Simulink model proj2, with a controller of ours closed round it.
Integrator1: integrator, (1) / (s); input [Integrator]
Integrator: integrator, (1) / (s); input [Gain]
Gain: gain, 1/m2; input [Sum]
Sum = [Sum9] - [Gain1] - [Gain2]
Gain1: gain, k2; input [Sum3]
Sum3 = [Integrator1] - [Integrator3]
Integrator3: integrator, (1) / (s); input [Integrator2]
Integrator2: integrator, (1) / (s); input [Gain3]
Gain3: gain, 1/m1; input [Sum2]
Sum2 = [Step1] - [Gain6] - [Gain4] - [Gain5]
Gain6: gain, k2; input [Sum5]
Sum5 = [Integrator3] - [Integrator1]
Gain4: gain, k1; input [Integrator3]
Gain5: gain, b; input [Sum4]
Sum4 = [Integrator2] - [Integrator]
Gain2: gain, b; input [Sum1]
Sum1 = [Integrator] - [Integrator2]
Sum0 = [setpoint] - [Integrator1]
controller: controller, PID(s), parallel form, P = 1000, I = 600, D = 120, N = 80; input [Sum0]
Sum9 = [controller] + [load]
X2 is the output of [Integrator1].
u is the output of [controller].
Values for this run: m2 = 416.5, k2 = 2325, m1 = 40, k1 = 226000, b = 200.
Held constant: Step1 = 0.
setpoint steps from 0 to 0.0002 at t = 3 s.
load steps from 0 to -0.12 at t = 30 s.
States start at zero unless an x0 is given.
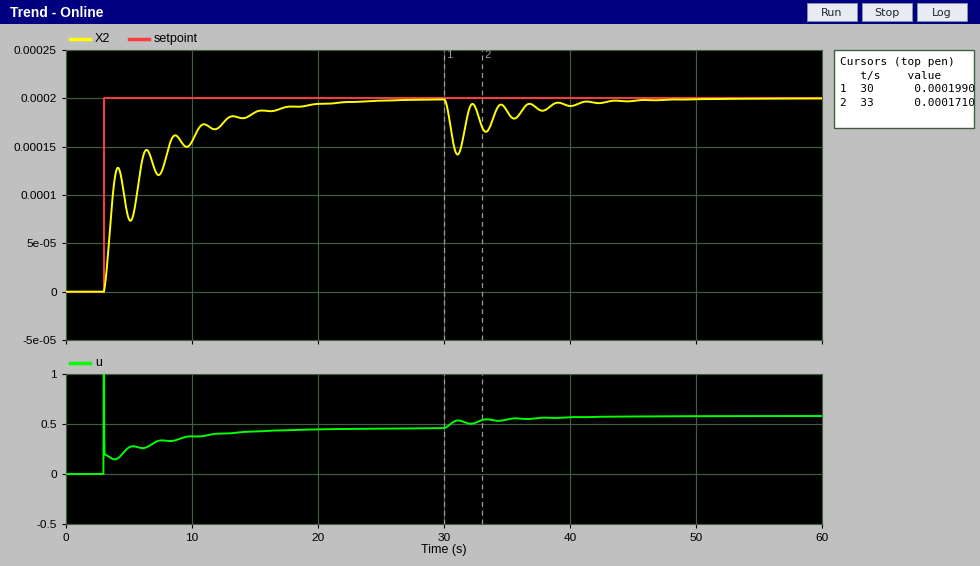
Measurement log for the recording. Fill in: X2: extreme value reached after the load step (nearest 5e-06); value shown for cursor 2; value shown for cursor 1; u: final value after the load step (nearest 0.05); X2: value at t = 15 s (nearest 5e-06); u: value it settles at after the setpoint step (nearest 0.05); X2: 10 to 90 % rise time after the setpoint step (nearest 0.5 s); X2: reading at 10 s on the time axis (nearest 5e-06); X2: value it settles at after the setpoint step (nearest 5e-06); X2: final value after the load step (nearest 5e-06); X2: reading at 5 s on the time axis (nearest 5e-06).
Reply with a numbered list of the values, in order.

1. 0.000140
2. 0.0001710
3. 0.0001990
4. 0.60
5. 0.000185
6. 0.45
7. 9.5 s
8. 0.000155
9. 0.000200
10. 0.000200
11. 0.000075
